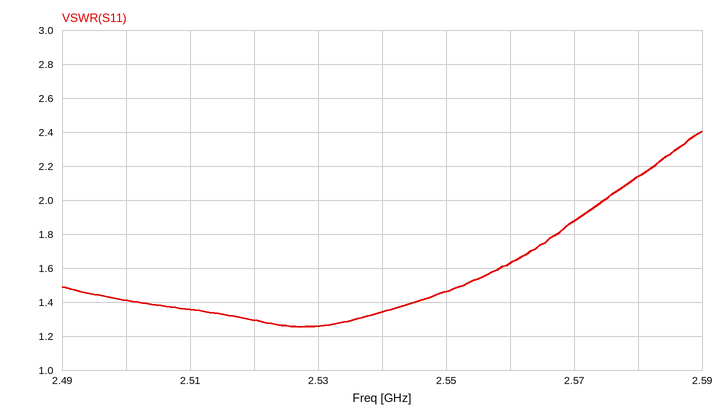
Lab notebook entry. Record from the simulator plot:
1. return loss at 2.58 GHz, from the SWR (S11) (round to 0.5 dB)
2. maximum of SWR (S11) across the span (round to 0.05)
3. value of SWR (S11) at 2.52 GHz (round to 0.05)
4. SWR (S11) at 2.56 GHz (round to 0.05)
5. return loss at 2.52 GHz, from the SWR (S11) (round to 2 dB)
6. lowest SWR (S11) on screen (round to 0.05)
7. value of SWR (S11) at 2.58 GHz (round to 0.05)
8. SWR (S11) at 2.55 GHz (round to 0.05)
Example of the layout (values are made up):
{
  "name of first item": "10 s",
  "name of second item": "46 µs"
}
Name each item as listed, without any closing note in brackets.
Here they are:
{
  "return loss at 2.58 GHz, from the SWR (S11)": "9.0 dB",
  "maximum of SWR (S11) across the span": "2.40",
  "value of SWR (S11) at 2.52 GHz": "1.30",
  "SWR (S11) at 2.56 GHz": "1.65",
  "return loss at 2.52 GHz, from the SWR (S11)": "18 dB",
  "lowest SWR (S11) on screen": "1.25",
  "value of SWR (S11) at 2.58 GHz": "2.15",
  "SWR (S11) at 2.55 GHz": "1.45"
}
